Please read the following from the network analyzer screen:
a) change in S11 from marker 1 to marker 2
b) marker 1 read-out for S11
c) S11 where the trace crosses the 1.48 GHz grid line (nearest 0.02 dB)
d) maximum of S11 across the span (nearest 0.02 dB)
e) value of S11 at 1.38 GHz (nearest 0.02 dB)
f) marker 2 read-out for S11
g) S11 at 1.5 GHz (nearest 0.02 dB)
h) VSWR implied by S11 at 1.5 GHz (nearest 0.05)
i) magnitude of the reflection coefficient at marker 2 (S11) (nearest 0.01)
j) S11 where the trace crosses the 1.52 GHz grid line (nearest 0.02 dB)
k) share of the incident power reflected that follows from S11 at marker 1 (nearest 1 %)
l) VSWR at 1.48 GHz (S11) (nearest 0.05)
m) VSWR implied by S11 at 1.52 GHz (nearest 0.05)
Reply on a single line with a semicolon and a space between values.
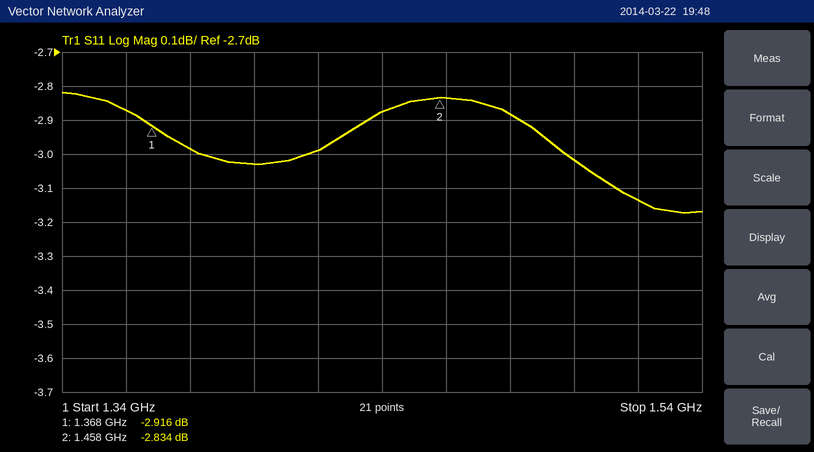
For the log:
0.082 dB; -2.916 dB; -2.88 dB; -2.82 dB; -2.98 dB; -2.834 dB; -3.02 dB; 5.80; 0.72; -3.14 dB; 51 %; 6.10; 5.60
